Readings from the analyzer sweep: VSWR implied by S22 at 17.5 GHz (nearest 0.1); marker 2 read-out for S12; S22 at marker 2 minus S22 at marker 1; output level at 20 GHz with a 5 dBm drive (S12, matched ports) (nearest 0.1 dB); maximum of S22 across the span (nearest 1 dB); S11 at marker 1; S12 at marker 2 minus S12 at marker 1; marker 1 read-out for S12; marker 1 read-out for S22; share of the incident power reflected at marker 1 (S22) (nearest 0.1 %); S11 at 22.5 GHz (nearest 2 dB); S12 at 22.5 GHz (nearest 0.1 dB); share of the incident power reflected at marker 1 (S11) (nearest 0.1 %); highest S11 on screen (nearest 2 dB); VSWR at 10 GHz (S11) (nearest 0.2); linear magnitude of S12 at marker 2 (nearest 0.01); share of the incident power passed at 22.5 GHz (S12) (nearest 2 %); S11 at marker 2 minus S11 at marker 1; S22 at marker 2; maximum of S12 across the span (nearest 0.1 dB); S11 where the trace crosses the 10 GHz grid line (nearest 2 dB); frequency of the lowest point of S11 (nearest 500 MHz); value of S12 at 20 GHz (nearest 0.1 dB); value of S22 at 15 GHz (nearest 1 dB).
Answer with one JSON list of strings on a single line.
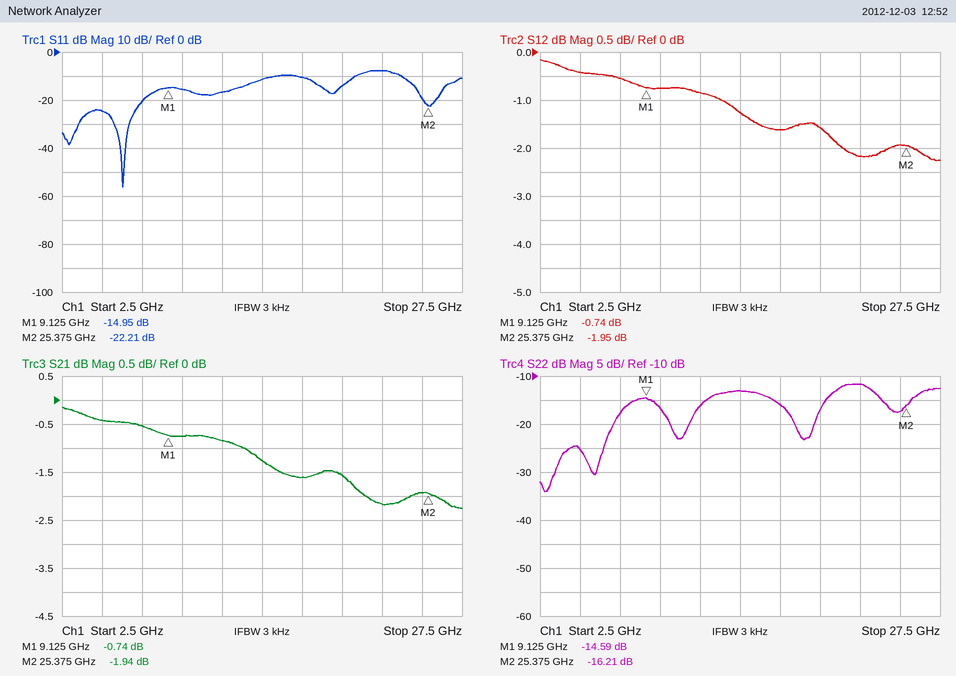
["1.4", "-1.95 dB", "-1.62 dB", "3.4 dBm", "-12 dB", "-14.95 dB", "-1.21 dB", "-0.74 dB", "-14.59 dB", "3.5 %", "-8 dB", "-2.2 dB", "3.2 %", "-8 dB", "1.4", "0.80", "60 %", "-7.26 dB", "-16.21 dB", "-0.2 dB", "-16 dB", "6.5 GHz", "-1.6 dB", "-13 dB"]
